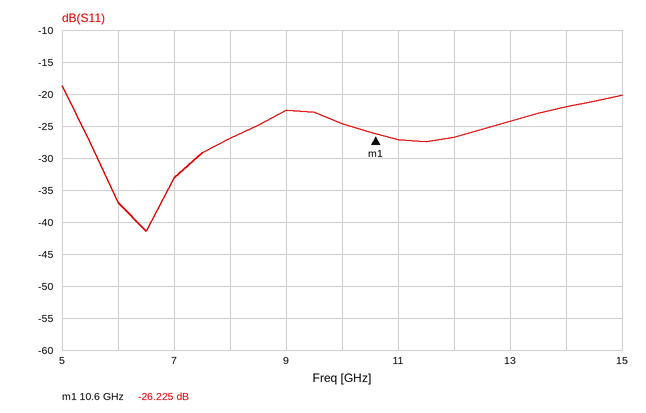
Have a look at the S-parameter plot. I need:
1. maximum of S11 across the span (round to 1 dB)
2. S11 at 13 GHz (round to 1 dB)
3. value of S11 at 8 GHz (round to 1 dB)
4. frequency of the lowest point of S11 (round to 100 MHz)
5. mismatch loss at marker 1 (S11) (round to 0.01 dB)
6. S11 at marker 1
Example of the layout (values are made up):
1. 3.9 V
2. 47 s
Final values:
1. -19 dB
2. -24 dB
3. -27 dB
4. 6.5 GHz
5. 0.01 dB
6. -26.225 dB
